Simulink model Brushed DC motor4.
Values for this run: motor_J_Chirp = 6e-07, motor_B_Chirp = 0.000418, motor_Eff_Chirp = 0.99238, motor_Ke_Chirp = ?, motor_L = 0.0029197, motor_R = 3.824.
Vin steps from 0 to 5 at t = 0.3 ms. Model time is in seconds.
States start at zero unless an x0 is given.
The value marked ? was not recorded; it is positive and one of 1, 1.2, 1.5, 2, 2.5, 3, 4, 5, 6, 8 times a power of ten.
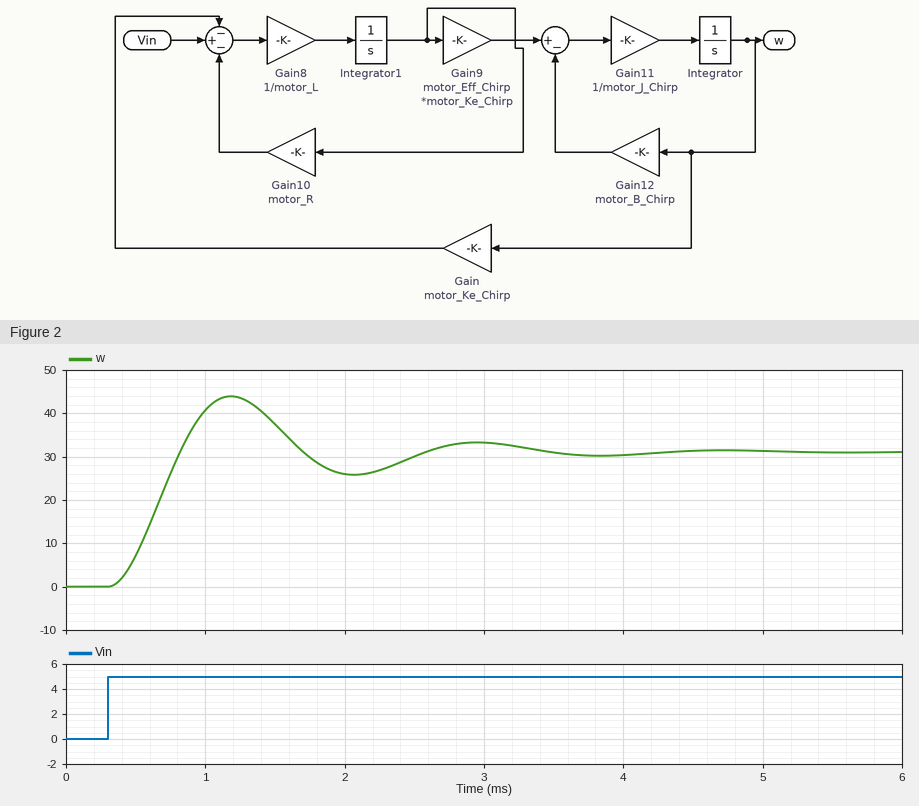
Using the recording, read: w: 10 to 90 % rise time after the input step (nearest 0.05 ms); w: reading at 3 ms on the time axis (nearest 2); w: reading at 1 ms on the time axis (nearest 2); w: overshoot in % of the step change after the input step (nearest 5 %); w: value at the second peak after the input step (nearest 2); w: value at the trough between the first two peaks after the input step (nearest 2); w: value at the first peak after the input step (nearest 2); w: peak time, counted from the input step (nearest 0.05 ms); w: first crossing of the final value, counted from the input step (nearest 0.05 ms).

0.35 ms
34
40
40 %
34
26
44
0.90 ms
0.50 ms
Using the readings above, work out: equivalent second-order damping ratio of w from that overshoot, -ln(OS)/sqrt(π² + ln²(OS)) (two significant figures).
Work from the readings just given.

0.28
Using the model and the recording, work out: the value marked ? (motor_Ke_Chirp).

0.15
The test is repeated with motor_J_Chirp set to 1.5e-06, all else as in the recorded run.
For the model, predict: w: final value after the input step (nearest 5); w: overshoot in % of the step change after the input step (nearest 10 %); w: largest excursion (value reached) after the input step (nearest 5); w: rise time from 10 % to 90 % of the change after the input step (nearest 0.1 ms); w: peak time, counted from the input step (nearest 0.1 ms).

30
30 %
40
0.6 ms
1.4 ms
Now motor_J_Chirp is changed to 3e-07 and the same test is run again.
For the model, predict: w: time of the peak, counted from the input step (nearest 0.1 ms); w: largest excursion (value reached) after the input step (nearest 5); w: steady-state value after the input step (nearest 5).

0.6 ms
45
30
